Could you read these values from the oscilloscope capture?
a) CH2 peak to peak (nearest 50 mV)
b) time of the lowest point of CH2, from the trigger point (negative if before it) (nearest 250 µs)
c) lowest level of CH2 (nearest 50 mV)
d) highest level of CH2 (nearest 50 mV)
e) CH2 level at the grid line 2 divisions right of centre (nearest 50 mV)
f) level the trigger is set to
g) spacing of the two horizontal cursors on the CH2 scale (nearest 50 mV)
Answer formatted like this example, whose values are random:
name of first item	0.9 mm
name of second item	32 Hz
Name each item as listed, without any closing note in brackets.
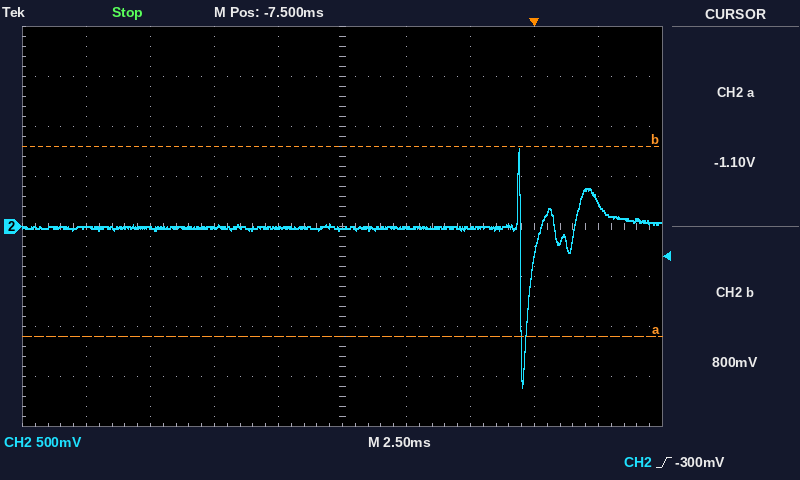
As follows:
CH2 peak to peak	2.40 V
time of the lowest point of CH2, from the trigger point (negative if before it)	-500 µs
lowest level of CH2	-1.60 V
highest level of CH2	800 mV
CH2 level at the grid line 2 divisions right of centre	0 mV
level the trigger is set to	-300 mV
spacing of the two horizontal cursors on the CH2 scale	1.90 V
